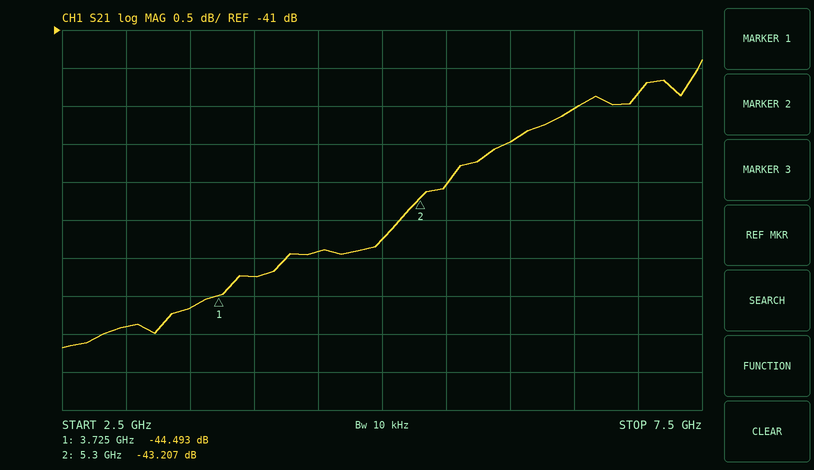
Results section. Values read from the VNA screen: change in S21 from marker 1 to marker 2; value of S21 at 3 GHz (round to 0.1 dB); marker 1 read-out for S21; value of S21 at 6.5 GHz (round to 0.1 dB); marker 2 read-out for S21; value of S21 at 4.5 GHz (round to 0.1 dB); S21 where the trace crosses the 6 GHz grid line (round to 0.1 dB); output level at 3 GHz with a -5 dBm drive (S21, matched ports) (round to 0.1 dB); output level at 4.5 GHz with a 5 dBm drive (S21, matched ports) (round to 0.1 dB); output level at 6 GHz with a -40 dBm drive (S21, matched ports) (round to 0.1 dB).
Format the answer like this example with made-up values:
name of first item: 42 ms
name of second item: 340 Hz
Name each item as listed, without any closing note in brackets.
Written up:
change in S21 from marker 1 to marker 2: 1.286 dB
value of S21 at 3 GHz: -44.9 dB
marker 1 read-out for S21: -44.493 dB
value of S21 at 6.5 GHz: -42.0 dB
marker 2 read-out for S21: -43.207 dB
value of S21 at 4.5 GHz: -43.9 dB
S21 where the trace crosses the 6 GHz grid line: -42.5 dB
output level at 3 GHz with a -5 dBm drive (S21, matched ports): -49.9 dBm
output level at 4.5 GHz with a 5 dBm drive (S21, matched ports): -38.9 dBm
output level at 6 GHz with a -40 dBm drive (S21, matched ports): -82.5 dBm
